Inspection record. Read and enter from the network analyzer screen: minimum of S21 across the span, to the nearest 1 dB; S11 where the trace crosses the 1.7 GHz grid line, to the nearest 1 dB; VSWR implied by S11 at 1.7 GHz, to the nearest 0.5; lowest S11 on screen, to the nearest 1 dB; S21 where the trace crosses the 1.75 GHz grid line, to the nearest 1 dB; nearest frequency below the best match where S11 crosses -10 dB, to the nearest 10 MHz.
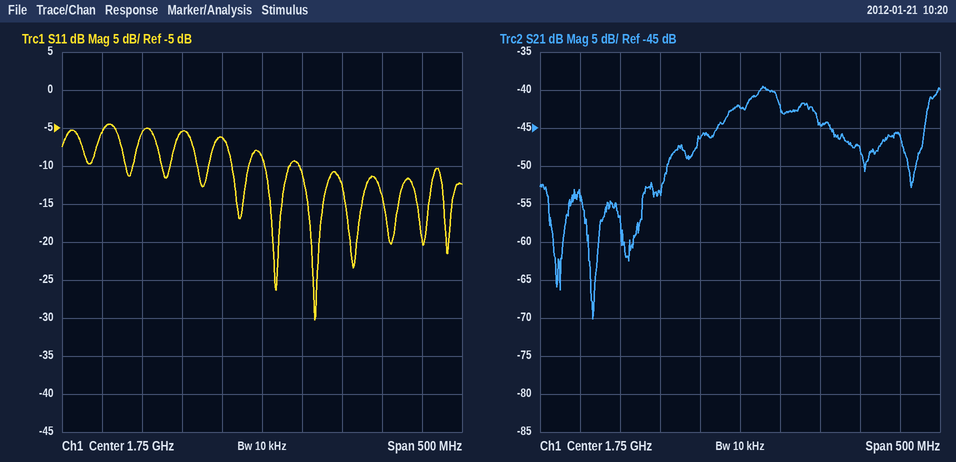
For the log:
-70 dB
-6 dB
3.0
-30 dB
-42 dB
1.80 GHz
